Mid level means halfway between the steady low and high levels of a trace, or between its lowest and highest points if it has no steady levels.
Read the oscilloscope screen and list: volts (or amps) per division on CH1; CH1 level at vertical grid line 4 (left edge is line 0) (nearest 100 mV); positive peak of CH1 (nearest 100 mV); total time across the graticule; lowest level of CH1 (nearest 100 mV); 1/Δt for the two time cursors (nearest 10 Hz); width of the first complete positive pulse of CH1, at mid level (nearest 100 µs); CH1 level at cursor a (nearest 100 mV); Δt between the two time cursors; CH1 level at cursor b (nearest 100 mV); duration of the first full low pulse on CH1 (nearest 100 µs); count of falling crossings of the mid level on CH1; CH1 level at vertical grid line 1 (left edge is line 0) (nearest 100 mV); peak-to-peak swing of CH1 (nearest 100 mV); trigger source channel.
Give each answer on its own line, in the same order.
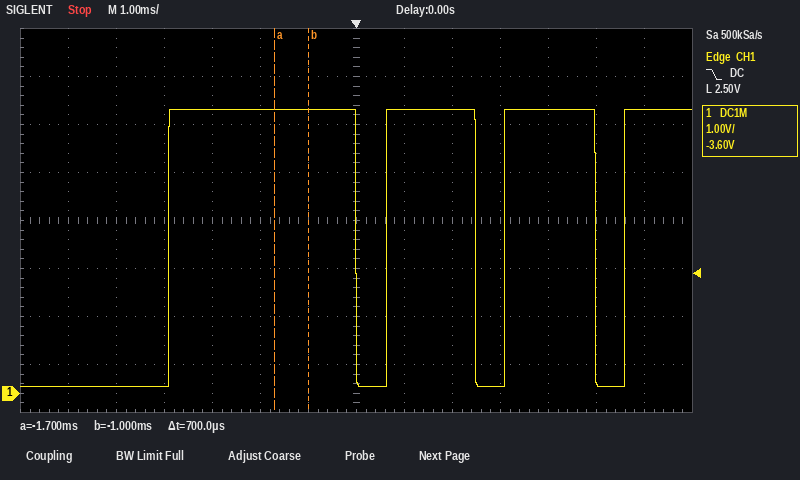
1 V
5.9 V
5.9 V
14 ms
100 mV
1.43 kHz
3.9 ms
5.9 V
700 µs
5.9 V
600 µs
3
100 mV
5.8 V
CH1
